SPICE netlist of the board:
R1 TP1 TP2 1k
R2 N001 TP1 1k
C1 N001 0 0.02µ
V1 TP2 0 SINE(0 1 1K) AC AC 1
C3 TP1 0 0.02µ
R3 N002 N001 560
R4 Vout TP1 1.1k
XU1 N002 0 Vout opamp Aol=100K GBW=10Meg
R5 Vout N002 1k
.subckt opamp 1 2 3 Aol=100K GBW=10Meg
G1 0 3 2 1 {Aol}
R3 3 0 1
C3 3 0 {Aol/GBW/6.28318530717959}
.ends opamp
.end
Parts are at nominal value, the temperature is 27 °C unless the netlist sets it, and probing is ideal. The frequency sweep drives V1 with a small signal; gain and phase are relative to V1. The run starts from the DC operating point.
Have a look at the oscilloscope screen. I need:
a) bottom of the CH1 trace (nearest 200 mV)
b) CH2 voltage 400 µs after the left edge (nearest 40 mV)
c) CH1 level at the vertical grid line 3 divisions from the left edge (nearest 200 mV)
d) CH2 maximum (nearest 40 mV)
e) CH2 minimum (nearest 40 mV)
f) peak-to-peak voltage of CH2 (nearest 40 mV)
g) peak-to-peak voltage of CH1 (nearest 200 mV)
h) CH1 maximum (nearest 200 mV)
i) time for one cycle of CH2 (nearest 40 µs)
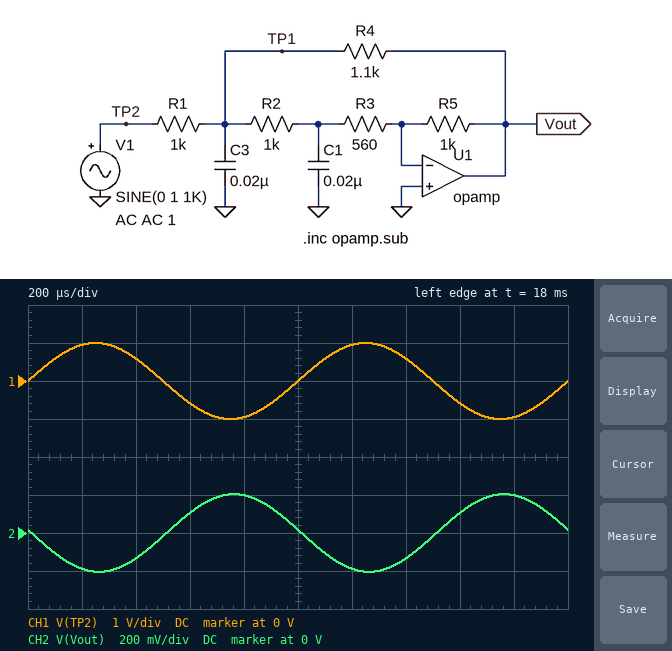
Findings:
-1.0 V
-120 mV
-600 mV
200 mV
-200 mV
400 mV
2.0 V
1.0 V
1.00 ms
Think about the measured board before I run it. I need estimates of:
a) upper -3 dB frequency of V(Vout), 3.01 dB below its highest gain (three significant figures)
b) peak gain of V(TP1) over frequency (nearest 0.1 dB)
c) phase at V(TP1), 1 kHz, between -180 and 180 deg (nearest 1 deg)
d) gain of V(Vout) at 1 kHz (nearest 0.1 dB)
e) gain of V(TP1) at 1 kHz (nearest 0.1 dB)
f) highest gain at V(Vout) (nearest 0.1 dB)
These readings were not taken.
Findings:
16.0 kHz
-9.9 dB
-2 deg
-13.8 dB
-9.9 dB
-13.8 dB
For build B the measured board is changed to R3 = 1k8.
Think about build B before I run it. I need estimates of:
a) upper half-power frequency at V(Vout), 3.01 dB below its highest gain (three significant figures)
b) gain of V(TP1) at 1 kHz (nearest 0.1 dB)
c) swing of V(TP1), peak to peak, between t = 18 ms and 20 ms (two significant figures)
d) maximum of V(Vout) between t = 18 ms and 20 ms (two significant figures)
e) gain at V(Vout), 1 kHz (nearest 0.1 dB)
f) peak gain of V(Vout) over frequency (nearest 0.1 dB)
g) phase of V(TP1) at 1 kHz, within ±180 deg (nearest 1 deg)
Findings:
8.86 kHz
-8.3 dB
770 mV
140 mV
-17.3 dB
-17.2 dB
-3 deg
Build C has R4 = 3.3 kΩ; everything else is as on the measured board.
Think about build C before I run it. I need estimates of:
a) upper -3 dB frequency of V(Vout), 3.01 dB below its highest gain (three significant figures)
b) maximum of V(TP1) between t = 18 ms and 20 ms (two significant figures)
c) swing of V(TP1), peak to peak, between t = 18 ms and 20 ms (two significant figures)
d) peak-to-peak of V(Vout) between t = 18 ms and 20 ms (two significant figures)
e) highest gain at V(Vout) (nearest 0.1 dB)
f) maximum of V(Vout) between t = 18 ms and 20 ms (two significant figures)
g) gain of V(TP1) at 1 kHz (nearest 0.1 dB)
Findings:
11.8 kHz
470 mV
930 mV
600 mV
-10.5 dB
300 mV
-6.6 dB
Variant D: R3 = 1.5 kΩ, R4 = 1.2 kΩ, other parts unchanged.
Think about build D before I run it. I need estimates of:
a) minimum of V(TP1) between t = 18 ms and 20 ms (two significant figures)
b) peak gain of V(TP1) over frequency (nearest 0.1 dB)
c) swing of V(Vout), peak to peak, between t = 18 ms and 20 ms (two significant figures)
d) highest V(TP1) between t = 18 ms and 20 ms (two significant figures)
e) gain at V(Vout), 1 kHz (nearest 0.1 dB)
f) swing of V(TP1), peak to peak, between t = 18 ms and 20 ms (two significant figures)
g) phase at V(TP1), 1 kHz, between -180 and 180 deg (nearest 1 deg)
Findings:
-390 mV
-8.2 dB
310 mV
390 mV
-16.2 dB
780 mV
-3 deg
